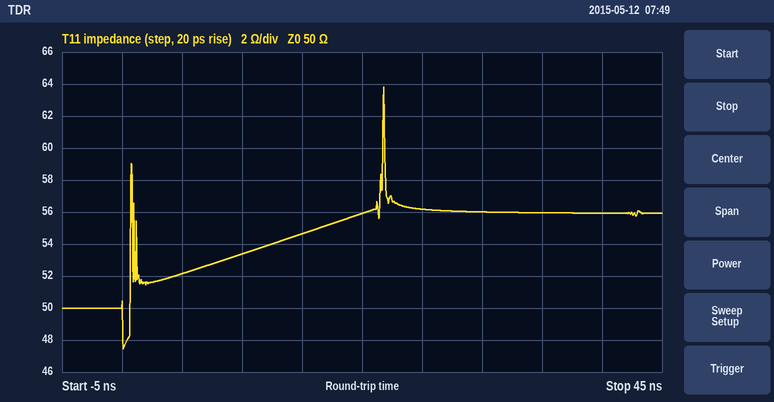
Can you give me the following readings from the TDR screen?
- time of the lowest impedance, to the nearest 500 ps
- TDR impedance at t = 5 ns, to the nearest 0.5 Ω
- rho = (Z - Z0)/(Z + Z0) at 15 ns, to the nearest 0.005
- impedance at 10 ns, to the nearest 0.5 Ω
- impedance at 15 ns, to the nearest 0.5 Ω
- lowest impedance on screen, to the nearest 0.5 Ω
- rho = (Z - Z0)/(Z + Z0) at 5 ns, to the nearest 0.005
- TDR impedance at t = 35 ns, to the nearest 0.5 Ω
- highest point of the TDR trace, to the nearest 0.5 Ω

0.0 ns
52.0 Ω
+0.045
53.5 Ω
54.5 Ω
47.5 Ω
+0.020
56.0 Ω
64.0 Ω
